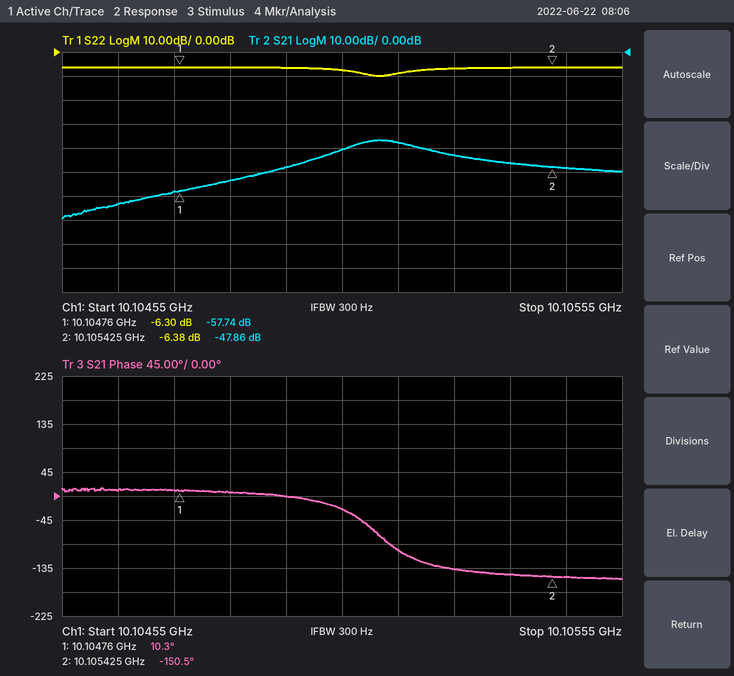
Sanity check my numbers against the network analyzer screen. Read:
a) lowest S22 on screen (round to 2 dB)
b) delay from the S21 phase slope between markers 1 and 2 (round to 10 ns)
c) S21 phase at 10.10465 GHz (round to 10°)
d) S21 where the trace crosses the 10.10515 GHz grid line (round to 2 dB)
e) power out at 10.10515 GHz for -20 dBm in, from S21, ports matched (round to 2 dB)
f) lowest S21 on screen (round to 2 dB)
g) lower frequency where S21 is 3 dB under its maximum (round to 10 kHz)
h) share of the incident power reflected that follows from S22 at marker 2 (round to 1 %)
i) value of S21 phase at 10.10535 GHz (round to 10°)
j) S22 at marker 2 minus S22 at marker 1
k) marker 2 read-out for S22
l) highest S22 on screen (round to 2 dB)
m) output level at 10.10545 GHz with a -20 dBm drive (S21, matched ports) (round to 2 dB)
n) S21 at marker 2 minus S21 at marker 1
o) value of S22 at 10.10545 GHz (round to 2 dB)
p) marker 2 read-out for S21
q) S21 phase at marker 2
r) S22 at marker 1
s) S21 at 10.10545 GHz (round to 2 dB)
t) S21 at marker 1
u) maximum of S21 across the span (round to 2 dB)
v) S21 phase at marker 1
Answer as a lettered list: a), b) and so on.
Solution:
a) -10 dB
b) 670 ns
c) 10°
d) -38 dB
e) -58 dBm
f) -70 dB
g) 10.10506 GHz
h) 23 %
i) -150°
j) -0.08 dB
k) -6.38 dB
l) -6 dB
m) -68 dBm
n) 9.88 dB
o) -6 dB
p) -47.86 dB
q) -150.5°
r) -6.30 dB
s) -48 dB
t) -57.74 dB
u) -36 dB
v) 10.3°
